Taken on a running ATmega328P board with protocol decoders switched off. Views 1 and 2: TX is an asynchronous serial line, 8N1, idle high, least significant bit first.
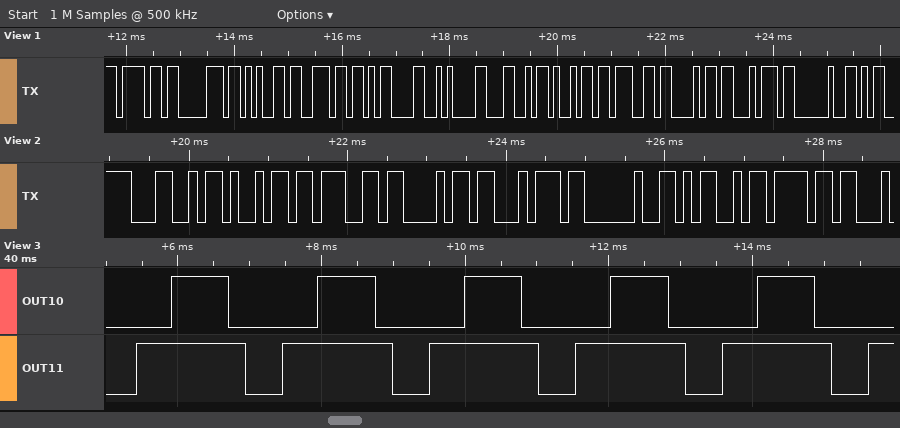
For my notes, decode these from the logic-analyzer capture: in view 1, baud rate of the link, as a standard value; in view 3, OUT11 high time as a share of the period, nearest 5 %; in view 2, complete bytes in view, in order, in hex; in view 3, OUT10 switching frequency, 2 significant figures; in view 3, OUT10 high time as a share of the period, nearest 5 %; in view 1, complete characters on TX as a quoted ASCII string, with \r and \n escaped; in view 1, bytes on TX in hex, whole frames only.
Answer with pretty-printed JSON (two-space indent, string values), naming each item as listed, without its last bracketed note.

{
  "in view 1, baud rate of the link, as a standard value": "9600 baud",
  "in view 3, OUT11 high time as a share of the period, nearest 5 %": "75 %",
  "in view 2, complete bytes in view, in order, in hex": "4C 69 67 68 74 20 4D 6F",
  "in view 3, OUT10 switching frequency, 2 significant figures": "490 Hz",
  "in view 3, OUT10 high time as a share of the period, nearest 5 %": "40 %",
  "in view 1, complete characters on TX as a quoted ASCII string, with \\r and \\n escaped": "\"open\\r\\nLight \"",
  "in view 1, bytes on TX in hex, whole frames only": "6F 70 65 6E 0D 0A 4C 69 67 68 74 20"
}
